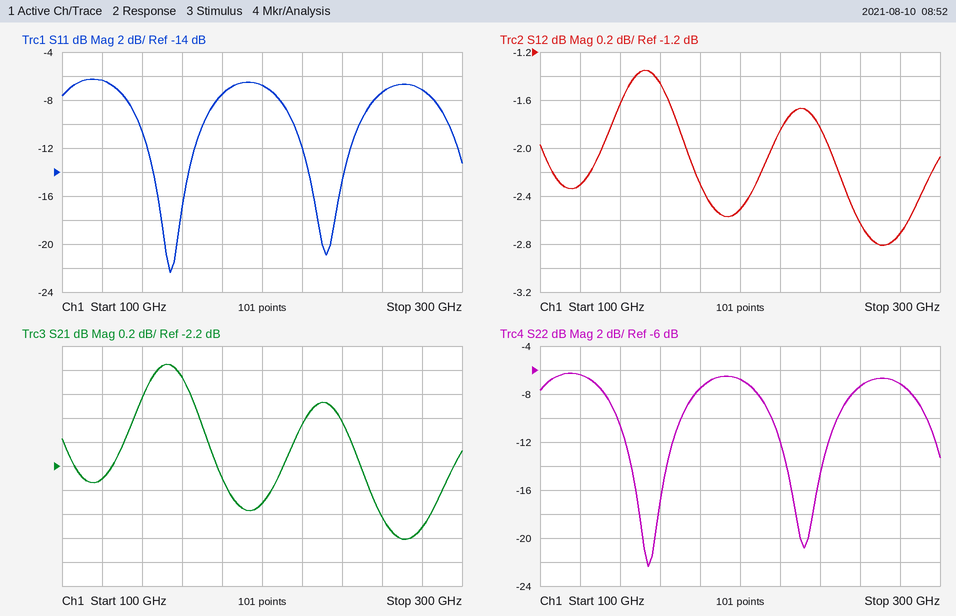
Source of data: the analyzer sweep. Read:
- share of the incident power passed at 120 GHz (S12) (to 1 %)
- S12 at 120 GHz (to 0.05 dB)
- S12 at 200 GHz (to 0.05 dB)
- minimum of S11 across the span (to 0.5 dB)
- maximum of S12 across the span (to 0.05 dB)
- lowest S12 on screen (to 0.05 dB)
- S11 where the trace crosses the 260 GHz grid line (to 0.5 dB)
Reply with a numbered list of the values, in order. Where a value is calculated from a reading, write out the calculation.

1. 10^(-2.3/10) ≈ 59 %
2. -2.30 dB
3. -2.50 dB
4. -22.5 dB
5. -1.35 dB
6. -2.80 dB
7. -7.5 dB
